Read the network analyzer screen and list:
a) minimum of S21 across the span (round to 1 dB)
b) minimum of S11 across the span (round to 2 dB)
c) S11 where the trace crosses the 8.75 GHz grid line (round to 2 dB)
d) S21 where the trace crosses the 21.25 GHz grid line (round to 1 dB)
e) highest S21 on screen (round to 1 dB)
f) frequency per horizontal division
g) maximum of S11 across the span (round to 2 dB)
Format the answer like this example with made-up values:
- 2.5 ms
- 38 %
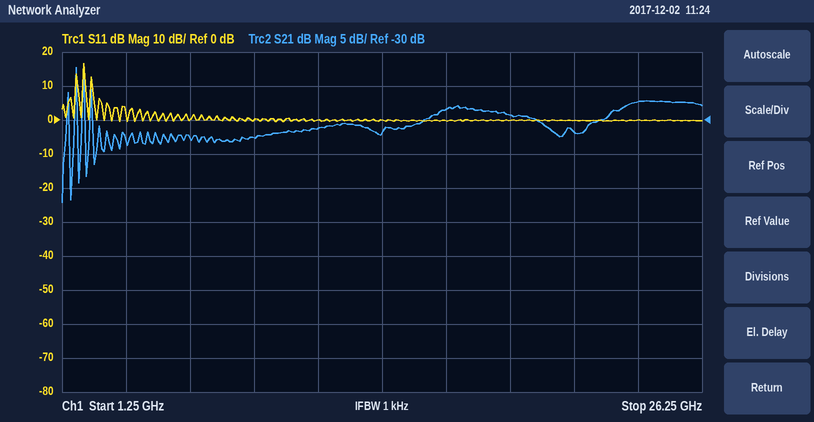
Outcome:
- -42 dB
- 0 dB
- 0 dB
- -32 dB
- -22 dB
- 2.5 GHz
- 16 dB
